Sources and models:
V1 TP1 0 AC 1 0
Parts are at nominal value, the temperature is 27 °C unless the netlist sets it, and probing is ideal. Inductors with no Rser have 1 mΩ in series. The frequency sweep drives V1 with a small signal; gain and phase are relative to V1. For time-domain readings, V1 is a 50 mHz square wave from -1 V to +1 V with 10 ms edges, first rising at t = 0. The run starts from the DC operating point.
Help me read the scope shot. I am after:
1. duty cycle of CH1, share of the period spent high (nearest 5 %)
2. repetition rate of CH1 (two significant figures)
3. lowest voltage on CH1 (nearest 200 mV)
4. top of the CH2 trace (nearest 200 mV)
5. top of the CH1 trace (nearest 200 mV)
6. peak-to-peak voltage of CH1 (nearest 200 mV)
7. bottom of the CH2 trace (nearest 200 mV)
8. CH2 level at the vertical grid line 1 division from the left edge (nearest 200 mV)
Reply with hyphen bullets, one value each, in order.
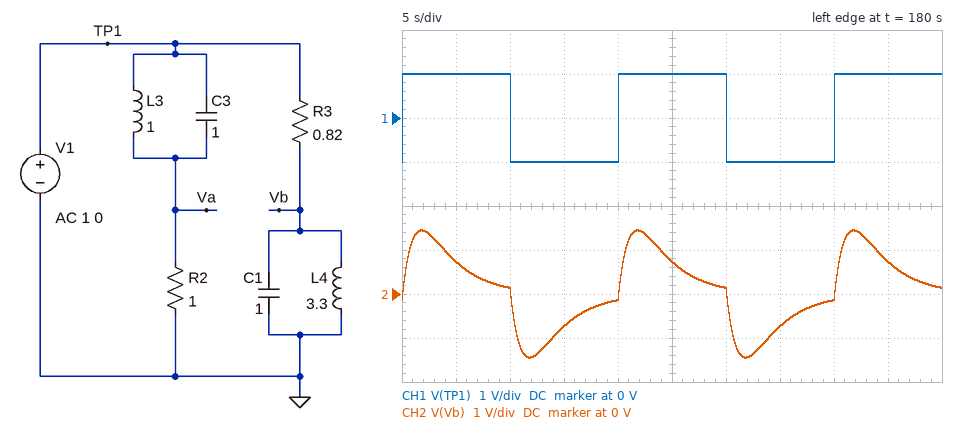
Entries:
- 50 %
- 50 mHz
- -1.0 V
- 1.4 V
- 1.0 V
- 2.0 V
- -1.4 V
- 800 mV
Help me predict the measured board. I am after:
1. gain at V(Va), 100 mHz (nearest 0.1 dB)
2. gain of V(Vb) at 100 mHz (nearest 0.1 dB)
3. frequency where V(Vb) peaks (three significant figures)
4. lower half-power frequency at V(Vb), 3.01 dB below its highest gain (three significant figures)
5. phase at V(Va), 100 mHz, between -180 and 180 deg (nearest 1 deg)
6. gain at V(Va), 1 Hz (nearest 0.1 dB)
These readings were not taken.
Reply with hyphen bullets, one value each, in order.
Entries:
- -3.2 dB
- -0.1 dB
- 87.7 mHz
- 33.7 mHz
- -46 deg
- -0.1 dB
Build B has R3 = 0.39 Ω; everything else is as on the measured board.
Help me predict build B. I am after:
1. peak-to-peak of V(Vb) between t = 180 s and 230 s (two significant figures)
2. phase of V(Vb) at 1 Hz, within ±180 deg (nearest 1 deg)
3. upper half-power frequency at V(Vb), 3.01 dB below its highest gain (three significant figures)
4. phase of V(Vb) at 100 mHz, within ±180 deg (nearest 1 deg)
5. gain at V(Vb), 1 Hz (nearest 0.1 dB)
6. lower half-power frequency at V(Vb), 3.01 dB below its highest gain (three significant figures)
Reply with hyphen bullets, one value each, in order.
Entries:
- 2.7 V
- -68 deg
- 426 mHz
- -3 deg
- -8.4 dB
- 18.1 mHz
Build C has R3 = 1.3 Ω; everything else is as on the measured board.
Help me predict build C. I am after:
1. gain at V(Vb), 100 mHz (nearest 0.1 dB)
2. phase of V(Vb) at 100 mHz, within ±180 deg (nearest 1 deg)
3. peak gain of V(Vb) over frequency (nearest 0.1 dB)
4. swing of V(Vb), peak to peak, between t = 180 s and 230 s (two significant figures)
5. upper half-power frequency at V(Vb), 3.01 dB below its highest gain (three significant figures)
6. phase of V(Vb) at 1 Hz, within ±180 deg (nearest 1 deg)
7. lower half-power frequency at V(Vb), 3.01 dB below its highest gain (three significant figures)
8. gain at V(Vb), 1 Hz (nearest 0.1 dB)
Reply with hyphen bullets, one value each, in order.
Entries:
- -0.2 dB
- -11 deg
- 0 dB
- 2.6 V
- 168 mHz
- -83 deg
- 45.7 mHz
- -18.2 dB
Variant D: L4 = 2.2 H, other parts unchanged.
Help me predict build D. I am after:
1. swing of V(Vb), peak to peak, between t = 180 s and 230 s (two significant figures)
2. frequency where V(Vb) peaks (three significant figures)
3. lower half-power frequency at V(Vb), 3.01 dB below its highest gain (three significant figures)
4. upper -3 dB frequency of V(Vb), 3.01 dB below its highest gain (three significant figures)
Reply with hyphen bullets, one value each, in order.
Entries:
- 2.8 V
- 107 mHz
- 47.7 mHz
- 242 mHz
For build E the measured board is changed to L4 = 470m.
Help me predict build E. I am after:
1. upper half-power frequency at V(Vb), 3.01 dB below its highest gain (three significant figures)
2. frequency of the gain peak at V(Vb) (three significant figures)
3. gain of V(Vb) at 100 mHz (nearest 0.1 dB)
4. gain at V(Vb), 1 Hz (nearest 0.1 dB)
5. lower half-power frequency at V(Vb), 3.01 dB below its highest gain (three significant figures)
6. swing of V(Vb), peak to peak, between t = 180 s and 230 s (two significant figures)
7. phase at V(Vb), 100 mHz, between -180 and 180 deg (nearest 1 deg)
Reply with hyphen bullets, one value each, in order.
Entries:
- 349 mHz
- 232 mHz
- -7.9 dB
- -13.9 dB
- 155 mHz
- 2.0 V
- 66 deg
